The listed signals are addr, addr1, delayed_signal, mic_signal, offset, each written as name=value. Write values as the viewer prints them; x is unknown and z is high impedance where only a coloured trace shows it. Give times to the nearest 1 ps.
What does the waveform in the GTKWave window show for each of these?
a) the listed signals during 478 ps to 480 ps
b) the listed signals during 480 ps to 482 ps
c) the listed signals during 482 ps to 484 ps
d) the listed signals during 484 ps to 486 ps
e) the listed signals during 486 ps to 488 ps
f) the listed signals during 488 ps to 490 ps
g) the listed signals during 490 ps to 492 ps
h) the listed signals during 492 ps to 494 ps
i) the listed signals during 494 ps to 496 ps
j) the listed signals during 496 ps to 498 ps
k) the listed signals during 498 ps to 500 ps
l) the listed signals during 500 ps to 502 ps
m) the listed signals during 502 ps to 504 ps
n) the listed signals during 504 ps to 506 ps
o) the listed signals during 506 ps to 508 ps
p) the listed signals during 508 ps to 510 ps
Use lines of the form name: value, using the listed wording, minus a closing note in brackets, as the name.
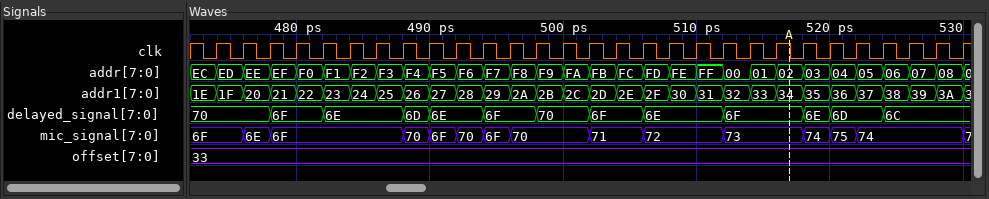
the listed signals during 478 ps to 480 ps: addr=EF, addr1=21, delayed_signal=6F, mic_signal=6F, offset=33
the listed signals during 480 ps to 482 ps: addr=F0, addr1=22, delayed_signal=6F, mic_signal=6F, offset=33
the listed signals during 482 ps to 484 ps: addr=F1, addr1=23, delayed_signal=6E, mic_signal=6F, offset=33
the listed signals during 484 ps to 486 ps: addr=F2, addr1=24, delayed_signal=6E, mic_signal=6F, offset=33
the listed signals during 486 ps to 488 ps: addr=F3, addr1=25, delayed_signal=6E, mic_signal=6F, offset=33
the listed signals during 488 ps to 490 ps: addr=F4, addr1=26, delayed_signal=6D, mic_signal=70, offset=33
the listed signals during 490 ps to 492 ps: addr=F5, addr1=27, delayed_signal=6E, mic_signal=6F, offset=33
the listed signals during 492 ps to 494 ps: addr=F6, addr1=28, delayed_signal=6E, mic_signal=70, offset=33
the listed signals during 494 ps to 496 ps: addr=F7, addr1=29, delayed_signal=6F, mic_signal=6F, offset=33
the listed signals during 496 ps to 498 ps: addr=F8, addr1=2A, delayed_signal=6F, mic_signal=70, offset=33
the listed signals during 498 ps to 500 ps: addr=F9, addr1=2B, delayed_signal=70, mic_signal=70, offset=33
the listed signals during 500 ps to 502 ps: addr=FA, addr1=2C, delayed_signal=70, mic_signal=70, offset=33
the listed signals during 502 ps to 504 ps: addr=FB, addr1=2D, delayed_signal=6F, mic_signal=71, offset=33
the listed signals during 504 ps to 506 ps: addr=FC, addr1=2E, delayed_signal=6F, mic_signal=71, offset=33
the listed signals during 506 ps to 508 ps: addr=FD, addr1=2F, delayed_signal=6E, mic_signal=72, offset=33
the listed signals during 508 ps to 510 ps: addr=FE, addr1=30, delayed_signal=6E, mic_signal=72, offset=33
